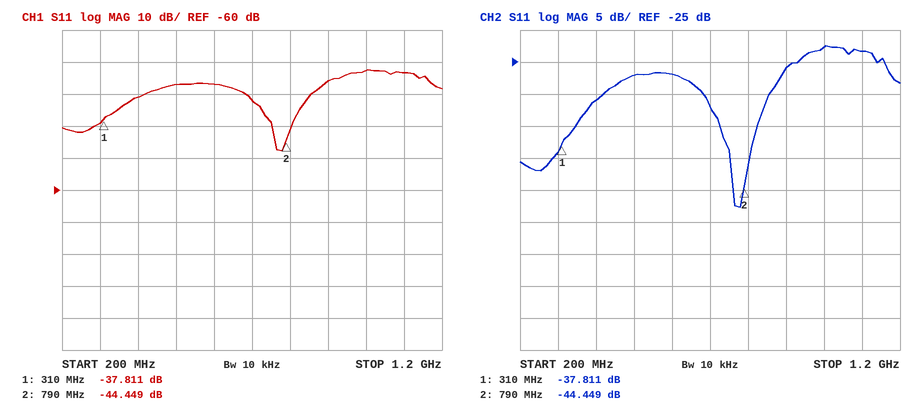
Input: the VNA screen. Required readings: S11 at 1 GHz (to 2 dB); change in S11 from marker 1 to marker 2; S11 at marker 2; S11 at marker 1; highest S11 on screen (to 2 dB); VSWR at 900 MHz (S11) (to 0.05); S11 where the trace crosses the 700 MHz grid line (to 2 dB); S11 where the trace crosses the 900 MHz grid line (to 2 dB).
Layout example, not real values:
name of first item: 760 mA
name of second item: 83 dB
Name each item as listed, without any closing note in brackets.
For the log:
S11 at 1 GHz: -22 dB
change in S11 from marker 1 to marker 2: -6.638 dB
S11 at marker 2: -44.449 dB
S11 at marker 1: -37.811 dB
highest S11 on screen: -22 dB
VSWR at 900 MHz (S11): 1.10
S11 where the trace crosses the 700 MHz grid line: -32 dB
S11 where the trace crosses the 900 MHz grid line: -26 dB
